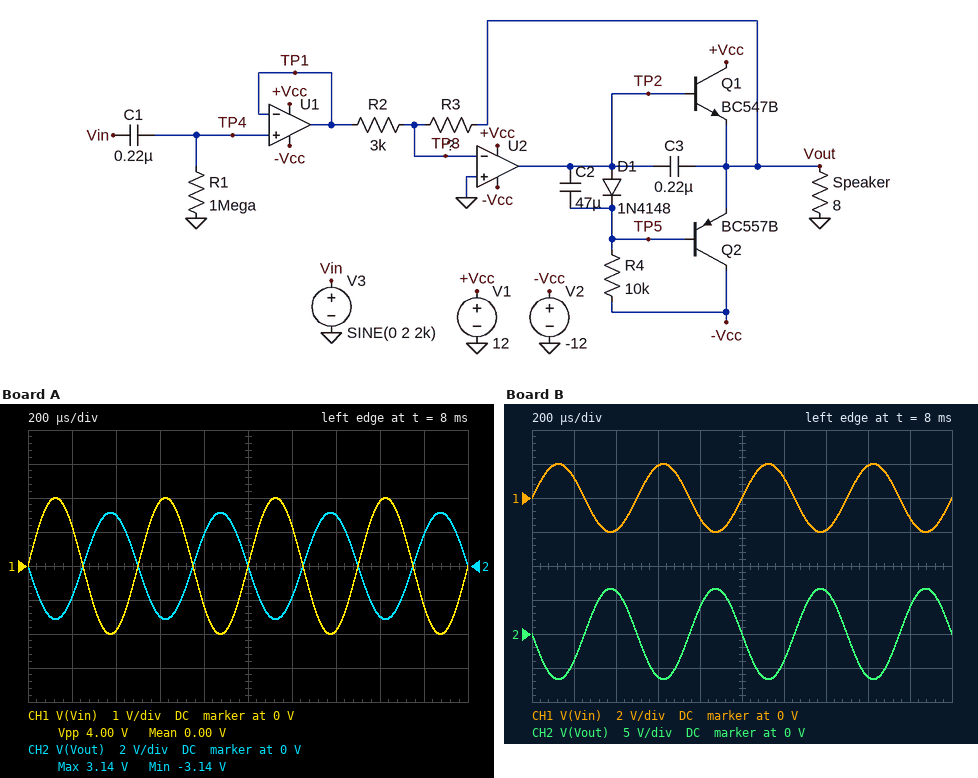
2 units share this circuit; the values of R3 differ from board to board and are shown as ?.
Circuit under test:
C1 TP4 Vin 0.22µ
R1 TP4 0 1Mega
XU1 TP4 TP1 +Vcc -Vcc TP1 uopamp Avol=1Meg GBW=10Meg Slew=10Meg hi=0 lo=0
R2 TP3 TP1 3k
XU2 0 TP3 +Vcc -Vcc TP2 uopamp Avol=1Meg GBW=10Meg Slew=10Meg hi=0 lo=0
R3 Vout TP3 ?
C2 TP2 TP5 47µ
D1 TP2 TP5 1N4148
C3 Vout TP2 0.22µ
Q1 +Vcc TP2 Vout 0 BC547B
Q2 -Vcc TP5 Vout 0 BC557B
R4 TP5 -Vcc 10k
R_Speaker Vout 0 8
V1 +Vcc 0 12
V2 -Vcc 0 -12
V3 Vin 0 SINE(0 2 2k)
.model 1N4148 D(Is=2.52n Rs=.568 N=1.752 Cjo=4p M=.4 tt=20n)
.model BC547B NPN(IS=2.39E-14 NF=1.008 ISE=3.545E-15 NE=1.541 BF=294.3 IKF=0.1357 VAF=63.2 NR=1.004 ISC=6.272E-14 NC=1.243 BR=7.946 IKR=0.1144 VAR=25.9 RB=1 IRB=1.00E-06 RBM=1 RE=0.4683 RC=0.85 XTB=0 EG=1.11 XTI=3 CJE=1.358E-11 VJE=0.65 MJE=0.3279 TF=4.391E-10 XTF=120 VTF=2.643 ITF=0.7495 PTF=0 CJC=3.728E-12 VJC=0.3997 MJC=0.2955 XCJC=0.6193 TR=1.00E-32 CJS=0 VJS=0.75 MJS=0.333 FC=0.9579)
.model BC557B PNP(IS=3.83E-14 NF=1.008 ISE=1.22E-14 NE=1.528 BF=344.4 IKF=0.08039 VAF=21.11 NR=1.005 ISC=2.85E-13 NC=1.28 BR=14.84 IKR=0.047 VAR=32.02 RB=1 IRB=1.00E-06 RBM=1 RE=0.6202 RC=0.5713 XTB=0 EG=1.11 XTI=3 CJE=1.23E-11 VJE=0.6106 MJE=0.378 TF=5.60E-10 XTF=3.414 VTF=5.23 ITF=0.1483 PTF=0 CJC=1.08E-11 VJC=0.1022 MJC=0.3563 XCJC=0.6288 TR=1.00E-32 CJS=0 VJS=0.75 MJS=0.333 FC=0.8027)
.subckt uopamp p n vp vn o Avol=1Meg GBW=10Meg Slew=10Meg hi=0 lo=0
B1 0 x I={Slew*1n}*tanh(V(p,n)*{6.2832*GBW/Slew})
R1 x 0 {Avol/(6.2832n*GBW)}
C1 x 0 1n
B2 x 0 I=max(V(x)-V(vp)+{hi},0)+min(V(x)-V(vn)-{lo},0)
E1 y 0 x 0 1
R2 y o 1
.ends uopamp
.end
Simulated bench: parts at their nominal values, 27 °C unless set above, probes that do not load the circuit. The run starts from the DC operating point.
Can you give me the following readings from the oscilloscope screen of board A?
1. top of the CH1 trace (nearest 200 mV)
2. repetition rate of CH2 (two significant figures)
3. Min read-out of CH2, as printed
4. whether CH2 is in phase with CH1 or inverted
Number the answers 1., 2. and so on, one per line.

1. 2.0 V
2. 2.0 kHz
3. -3.14 V
4. inverted
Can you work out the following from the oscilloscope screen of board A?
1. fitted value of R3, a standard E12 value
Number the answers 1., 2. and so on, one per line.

1. 4.7 kΩ
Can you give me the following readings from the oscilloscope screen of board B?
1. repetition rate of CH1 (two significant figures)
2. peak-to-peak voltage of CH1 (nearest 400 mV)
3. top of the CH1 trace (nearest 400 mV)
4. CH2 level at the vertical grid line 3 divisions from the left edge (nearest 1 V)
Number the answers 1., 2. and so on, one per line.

1. 2.0 kHz
2. 4.0 V
3. 2.0 V
4. -6 V
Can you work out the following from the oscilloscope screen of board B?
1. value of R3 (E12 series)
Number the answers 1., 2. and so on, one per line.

1. 10 kΩ
